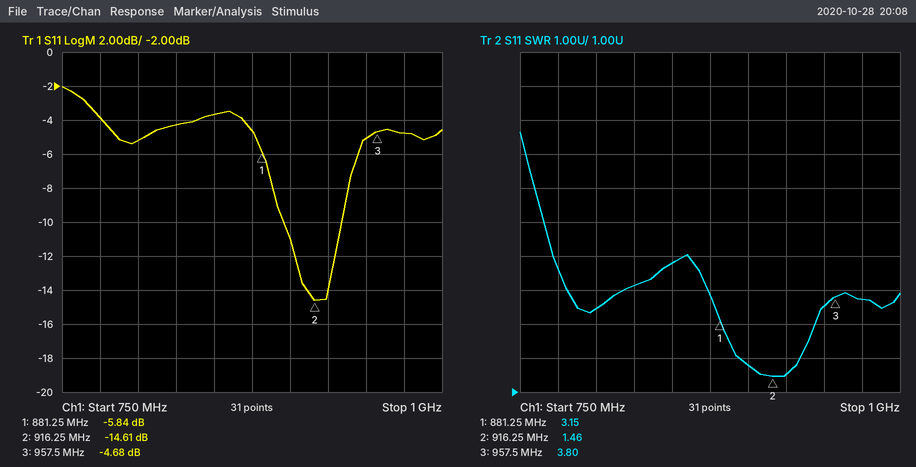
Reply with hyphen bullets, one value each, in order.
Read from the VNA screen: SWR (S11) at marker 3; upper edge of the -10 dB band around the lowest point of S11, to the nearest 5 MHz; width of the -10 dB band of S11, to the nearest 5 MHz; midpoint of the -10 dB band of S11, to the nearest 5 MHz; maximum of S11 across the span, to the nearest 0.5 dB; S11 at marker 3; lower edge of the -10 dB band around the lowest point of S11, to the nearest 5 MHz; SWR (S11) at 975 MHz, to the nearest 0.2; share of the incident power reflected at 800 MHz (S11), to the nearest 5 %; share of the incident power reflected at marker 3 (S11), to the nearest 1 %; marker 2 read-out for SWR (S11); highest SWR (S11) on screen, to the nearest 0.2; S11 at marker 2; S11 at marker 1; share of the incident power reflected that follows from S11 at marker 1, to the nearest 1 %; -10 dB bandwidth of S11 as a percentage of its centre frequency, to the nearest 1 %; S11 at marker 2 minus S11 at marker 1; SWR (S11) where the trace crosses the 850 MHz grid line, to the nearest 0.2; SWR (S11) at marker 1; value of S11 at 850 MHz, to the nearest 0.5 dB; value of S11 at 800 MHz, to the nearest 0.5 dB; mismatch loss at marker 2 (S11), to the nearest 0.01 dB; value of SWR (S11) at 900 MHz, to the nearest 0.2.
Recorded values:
- 3.80
- 935 MHz
- 40 MHz
- 915 MHz
- -2.0 dB
- -4.68 dB
- 895 MHz
- 3.8
- 30 %
- 34 %
- 1.46
- 8.6
- -14.61 dB
- -5.84 dB
- 26 %
- 4 %
- -8.77 dB
- 4.8
- 3.15
- -3.5 dB
- -5.0 dB
- 0.15 dB
- 1.8
